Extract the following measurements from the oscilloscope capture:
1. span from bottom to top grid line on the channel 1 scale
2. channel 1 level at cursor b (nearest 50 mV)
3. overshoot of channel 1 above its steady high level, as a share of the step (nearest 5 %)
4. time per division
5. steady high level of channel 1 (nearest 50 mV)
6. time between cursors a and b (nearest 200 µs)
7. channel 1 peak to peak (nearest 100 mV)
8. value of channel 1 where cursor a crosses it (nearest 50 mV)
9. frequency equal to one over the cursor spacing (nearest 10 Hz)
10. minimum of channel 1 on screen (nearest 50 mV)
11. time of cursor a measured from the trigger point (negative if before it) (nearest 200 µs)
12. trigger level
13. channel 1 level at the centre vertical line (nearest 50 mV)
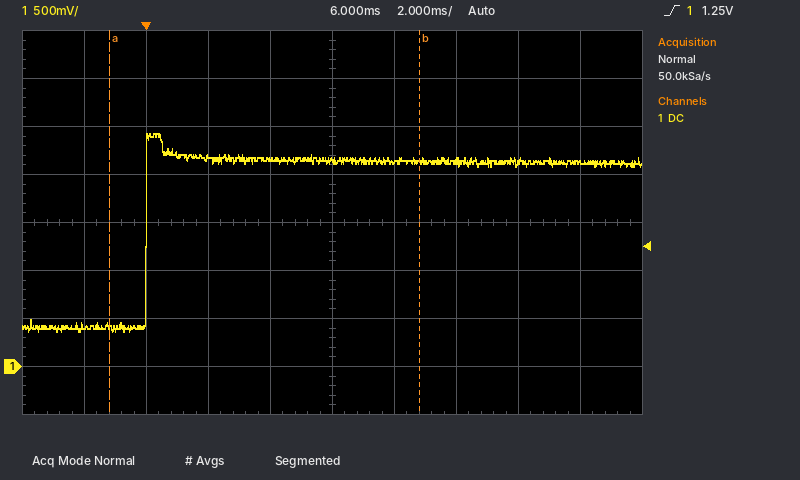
4 V
2.15 V
15 %
2 ms
2.15 V
10.0 ms
2.10 V
400 mV
100 Hz
350 mV
-1.2 ms
1.25 V
2.15 V
